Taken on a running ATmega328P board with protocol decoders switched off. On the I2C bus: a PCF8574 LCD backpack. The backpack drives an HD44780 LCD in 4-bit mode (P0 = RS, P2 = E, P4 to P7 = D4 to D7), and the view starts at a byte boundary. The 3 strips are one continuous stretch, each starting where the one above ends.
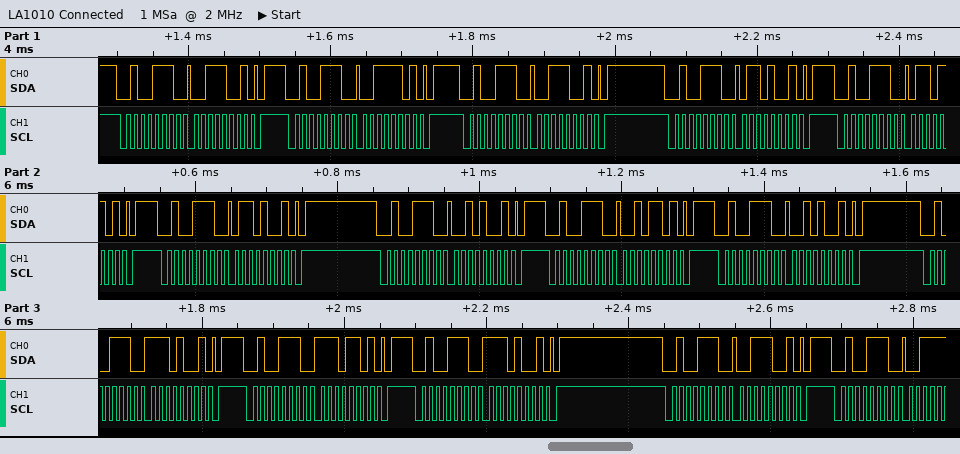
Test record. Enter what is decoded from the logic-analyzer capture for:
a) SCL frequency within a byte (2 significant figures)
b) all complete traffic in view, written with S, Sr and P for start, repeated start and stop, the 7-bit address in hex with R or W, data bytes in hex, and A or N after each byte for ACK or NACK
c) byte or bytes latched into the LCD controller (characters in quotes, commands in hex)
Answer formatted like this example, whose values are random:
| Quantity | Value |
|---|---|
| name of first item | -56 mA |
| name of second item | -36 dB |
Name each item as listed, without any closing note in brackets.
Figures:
| Quantity | Value |
|---|---|
| SCL frequency within a byte | 100 kHz |
| all complete traffic in view, written with S, Sr and P for start, repeated start and stop, the 7-bit address in hex with R or W, data bytes in hex, and A or N after each byte for ACK or NACK | S 27W A 39 A P S 27W A 3D A P S 27W A 39 A P S 27W A 69 A P S 27W A 6D A P S 27W A 69 A P S 27W A 29 A P S 27W A 2D A P S 27W A 29 A P S 27W A E9 A P S 27W A ED A P S 27W A E9 A P S 27W A 39 A P S 27W A |
| byte or bytes latched into the LCD controller | '6' '.' |
